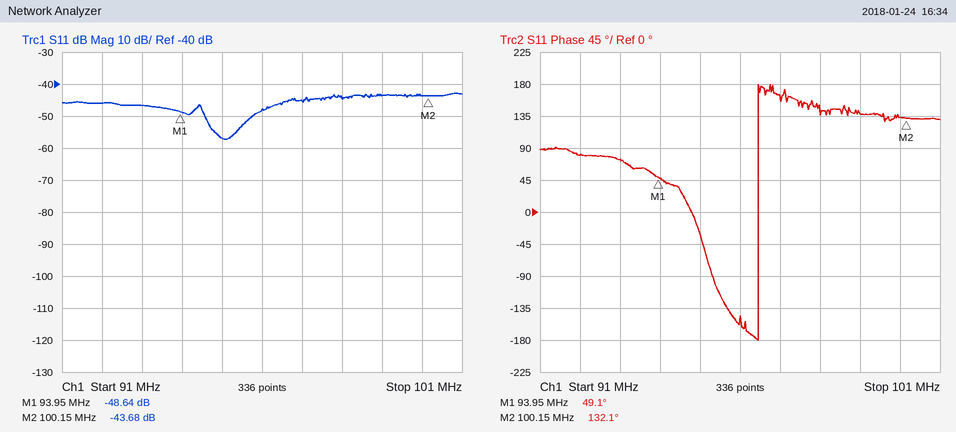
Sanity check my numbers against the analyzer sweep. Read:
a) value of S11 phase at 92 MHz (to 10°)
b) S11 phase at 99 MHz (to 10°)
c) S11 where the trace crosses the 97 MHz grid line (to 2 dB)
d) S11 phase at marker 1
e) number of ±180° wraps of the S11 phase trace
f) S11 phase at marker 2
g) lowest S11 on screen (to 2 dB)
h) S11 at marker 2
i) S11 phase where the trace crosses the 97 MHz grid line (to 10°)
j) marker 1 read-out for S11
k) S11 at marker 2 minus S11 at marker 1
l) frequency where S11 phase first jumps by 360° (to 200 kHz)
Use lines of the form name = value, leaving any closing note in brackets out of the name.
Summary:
value of S11 phase at 92 MHz = 80°
S11 phase at 99 MHz = 140°
S11 where the trace crosses the 97 MHz grid line = -46 dB
S11 phase at marker 1 = 49.1°
number of ±180° wraps of the S11 phase trace = 1
S11 phase at marker 2 = 132.1°
lowest S11 on screen = -58 dB
S11 at marker 2 = -43.68 dB
S11 phase where the trace crosses the 97 MHz grid line = 160°
marker 1 read-out for S11 = -48.64 dB
S11 at marker 2 minus S11 at marker 1 = 4.96 dB
frequency where S11 phase first jumps by 360° = 96.4 MHz
